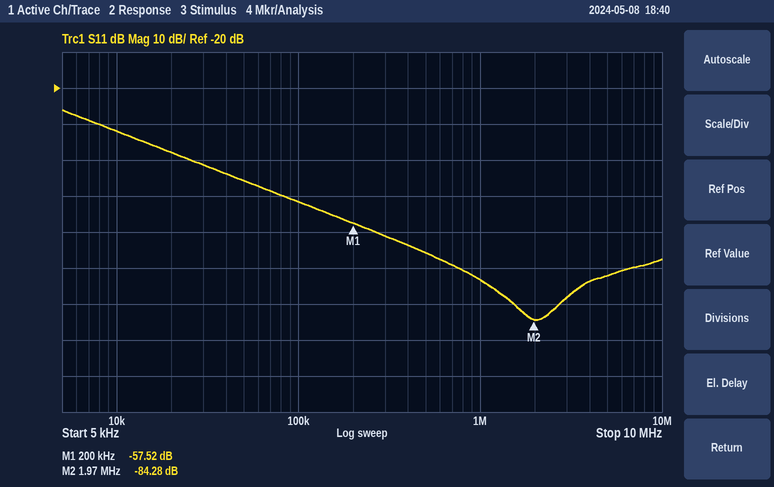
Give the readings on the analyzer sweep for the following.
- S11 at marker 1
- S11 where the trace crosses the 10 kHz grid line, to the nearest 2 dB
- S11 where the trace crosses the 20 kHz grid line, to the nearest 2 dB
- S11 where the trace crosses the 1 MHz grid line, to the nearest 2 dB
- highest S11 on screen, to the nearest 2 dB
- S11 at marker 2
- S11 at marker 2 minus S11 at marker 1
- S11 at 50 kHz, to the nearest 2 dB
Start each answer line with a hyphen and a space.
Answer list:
- -57.52 dB
- -32 dB
- -38 dB
- -74 dB
- -26 dB
- -84.28 dB
- -26.76 dB
- -46 dB
